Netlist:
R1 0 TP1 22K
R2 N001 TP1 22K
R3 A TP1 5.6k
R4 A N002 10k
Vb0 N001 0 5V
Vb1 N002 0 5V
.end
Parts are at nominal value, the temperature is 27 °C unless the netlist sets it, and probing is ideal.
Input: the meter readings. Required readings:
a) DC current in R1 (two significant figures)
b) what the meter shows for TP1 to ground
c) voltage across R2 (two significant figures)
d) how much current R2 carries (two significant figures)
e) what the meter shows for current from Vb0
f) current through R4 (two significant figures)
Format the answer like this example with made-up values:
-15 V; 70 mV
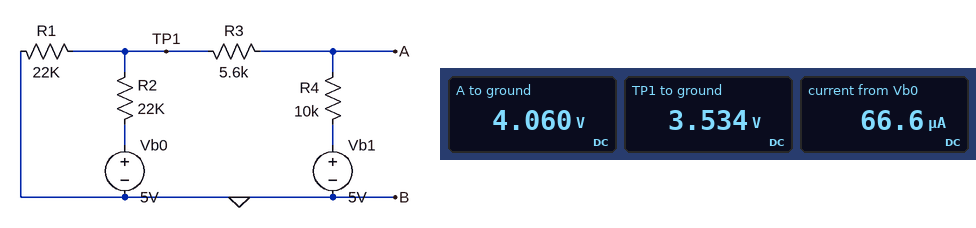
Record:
160 µA; 3.534 V; 1.5 V; 67 µA; 66.6 µA; 94 µA
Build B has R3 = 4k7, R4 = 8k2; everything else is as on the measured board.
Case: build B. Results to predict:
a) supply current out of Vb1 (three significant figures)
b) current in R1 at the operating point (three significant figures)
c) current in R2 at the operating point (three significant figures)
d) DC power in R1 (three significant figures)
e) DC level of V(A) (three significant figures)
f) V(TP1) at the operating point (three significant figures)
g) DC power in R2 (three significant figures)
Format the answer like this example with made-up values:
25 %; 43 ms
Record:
105 µA; 166 µA; 61.3 µA; 606 µW; 4.14 V; 3.65 V; 82.8 µW
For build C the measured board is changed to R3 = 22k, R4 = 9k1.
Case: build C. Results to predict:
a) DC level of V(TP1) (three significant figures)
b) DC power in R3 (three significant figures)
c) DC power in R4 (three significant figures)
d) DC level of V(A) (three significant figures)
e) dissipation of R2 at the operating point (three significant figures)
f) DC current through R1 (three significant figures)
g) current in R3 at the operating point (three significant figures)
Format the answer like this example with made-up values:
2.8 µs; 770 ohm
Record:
3.15 V; 77.6 µW; 32.1 µW; 4.46 V; 155 µW; 143 µA; 59.4 µA
